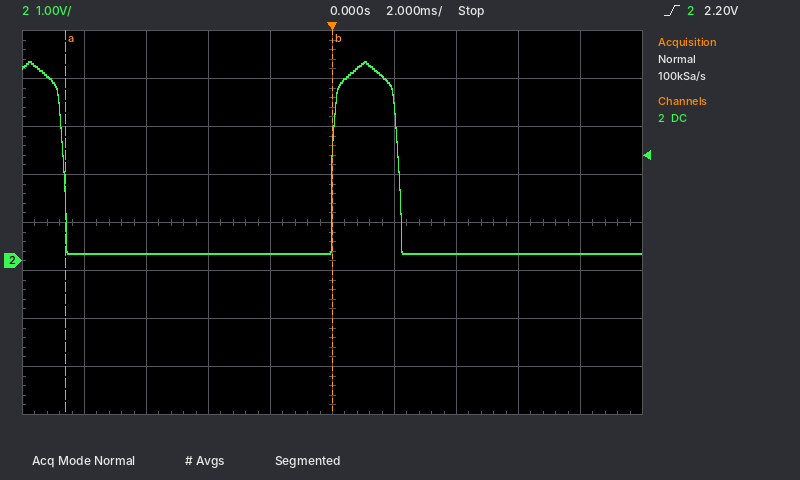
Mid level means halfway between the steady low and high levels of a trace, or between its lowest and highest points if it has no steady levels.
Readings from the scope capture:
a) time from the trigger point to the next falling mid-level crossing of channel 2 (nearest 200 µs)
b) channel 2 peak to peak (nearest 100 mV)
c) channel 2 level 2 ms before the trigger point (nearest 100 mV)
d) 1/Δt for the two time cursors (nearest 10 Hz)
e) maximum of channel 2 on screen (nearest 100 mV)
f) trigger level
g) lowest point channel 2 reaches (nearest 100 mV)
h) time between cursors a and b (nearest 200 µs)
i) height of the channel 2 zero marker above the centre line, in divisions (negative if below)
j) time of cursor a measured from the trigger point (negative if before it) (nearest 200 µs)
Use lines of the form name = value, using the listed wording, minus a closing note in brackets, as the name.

time from the trigger point to the next falling mid-level crossing of channel 2 = 2.2 ms
channel 2 peak to peak = 4.0 V
channel 2 level 2 ms before the trigger point = 200 mV
1/Δt for the two time cursors = 120 Hz
maximum of channel 2 on screen = 4.2 V
trigger level = 2.20 V
lowest point channel 2 reaches = 200 mV
time between cursors a and b = 8.6 ms
height of the channel 2 zero marker above the centre line, in divisions = -0.8 div
time of cursor a measured from the trigger point (negative if before it) = -8.6 ms
